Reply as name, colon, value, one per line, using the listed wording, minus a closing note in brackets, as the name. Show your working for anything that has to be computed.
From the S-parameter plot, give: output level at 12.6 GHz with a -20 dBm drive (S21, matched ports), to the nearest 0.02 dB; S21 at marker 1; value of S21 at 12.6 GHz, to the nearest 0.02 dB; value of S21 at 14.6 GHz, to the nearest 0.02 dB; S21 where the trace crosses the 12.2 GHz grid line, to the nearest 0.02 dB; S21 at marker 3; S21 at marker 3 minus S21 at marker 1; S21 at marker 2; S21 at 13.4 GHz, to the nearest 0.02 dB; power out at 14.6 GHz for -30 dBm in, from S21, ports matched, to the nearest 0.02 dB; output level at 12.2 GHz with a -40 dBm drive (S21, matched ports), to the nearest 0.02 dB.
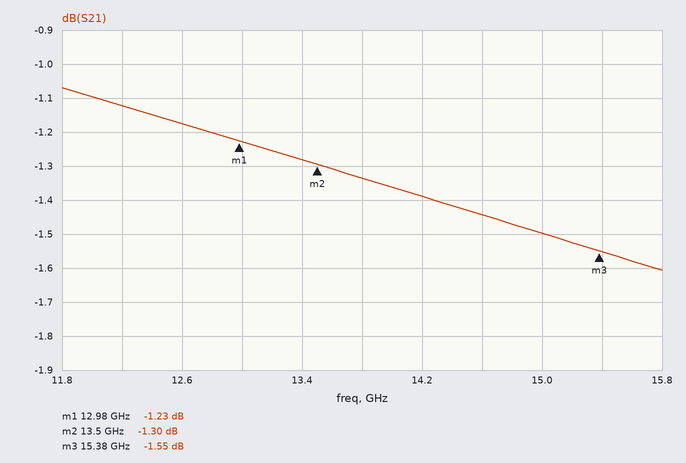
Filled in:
output level at 12.6 GHz with a -20 dBm drive (S21, matched ports), to the nearest 0.02 dB: -20 dBm + (-1.18 dB) = -21.18 dBm
S21 at marker 1: -1.23 dB
value of S21 at 12.6 GHz, to the nearest 0.02 dB: -1.18 dB
value of S21 at 14.6 GHz, to the nearest 0.02 dB: -1.44 dB
S21 where the trace crosses the 12.2 GHz grid line, to the nearest 0.02 dB: -1.12 dB
S21 at marker 3: -1.55 dB
S21 at marker 3 minus S21 at marker 1: -1.55 − (-1.23) = -0.32 dB
S21 at marker 2: -1.30 dB
S21 at 13.4 GHz, to the nearest 0.02 dB: -1.28 dB
power out at 14.6 GHz for -30 dBm in, from S21, ports matched, to the nearest 0.02 dB: -30 dBm + (-1.44 dB) = -31.44 dBm
output level at 12.2 GHz with a -40 dBm drive (S21, matched ports), to the nearest 0.02 dB: -40 dBm + (-1.12 dB) = -41.12 dBm
